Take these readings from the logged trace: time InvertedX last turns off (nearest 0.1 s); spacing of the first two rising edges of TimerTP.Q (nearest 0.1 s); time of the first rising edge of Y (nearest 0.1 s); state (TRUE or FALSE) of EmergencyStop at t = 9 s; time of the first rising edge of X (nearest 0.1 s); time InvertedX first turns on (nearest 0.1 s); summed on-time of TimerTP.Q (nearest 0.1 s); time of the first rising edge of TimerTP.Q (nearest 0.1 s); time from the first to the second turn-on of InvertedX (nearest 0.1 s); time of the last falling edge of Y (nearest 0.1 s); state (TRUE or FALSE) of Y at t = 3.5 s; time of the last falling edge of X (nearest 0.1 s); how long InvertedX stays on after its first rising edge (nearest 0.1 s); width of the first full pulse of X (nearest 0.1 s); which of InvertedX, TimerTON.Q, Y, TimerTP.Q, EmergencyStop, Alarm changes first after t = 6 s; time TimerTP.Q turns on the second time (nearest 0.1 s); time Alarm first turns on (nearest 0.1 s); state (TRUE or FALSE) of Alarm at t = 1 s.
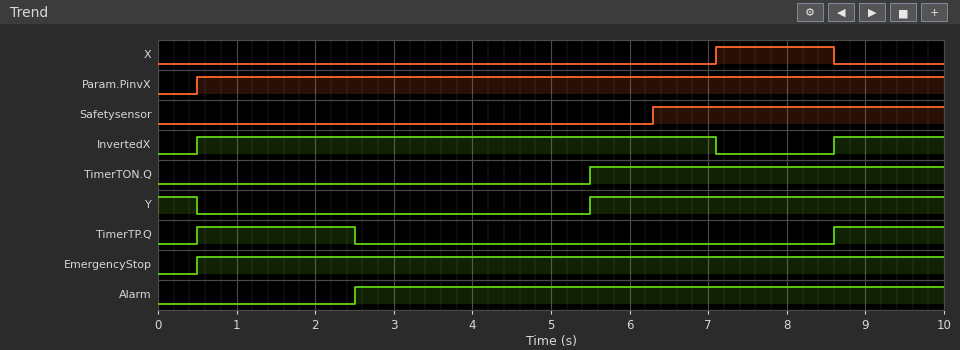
7.1 s
8.1 s
5.5 s
TRUE
7.1 s
0.5 s
3.4 s
0.5 s
8.1 s
0.5 s
FALSE
8.6 s
6.6 s
1.5 s
InvertedX
8.6 s
2.5 s
FALSE
